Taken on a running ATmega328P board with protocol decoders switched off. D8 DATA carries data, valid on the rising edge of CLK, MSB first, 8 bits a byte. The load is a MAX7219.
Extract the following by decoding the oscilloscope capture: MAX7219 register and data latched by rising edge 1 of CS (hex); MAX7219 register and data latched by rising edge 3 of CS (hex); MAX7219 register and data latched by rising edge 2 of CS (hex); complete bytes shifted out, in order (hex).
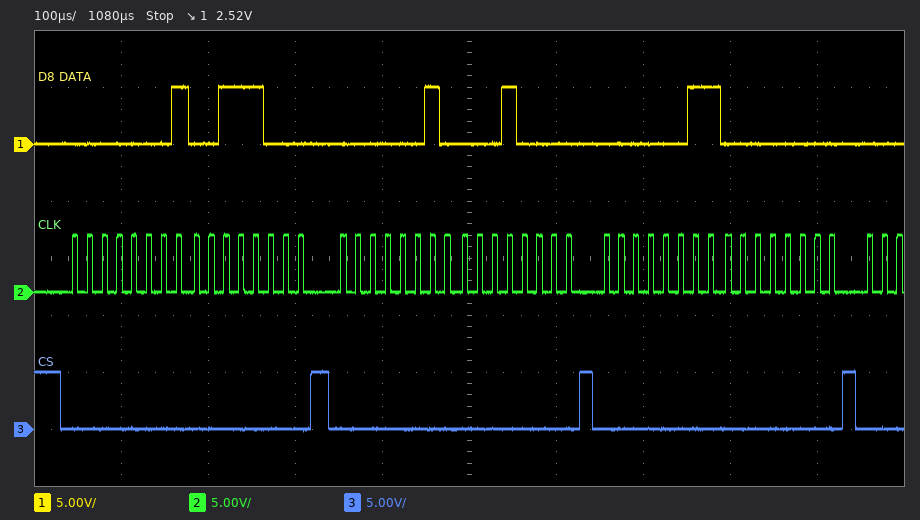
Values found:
register 0x1, data 0x38
register 0x3, data 0x00
register 0x2, data 0x10
01 38 02 10 03 00
